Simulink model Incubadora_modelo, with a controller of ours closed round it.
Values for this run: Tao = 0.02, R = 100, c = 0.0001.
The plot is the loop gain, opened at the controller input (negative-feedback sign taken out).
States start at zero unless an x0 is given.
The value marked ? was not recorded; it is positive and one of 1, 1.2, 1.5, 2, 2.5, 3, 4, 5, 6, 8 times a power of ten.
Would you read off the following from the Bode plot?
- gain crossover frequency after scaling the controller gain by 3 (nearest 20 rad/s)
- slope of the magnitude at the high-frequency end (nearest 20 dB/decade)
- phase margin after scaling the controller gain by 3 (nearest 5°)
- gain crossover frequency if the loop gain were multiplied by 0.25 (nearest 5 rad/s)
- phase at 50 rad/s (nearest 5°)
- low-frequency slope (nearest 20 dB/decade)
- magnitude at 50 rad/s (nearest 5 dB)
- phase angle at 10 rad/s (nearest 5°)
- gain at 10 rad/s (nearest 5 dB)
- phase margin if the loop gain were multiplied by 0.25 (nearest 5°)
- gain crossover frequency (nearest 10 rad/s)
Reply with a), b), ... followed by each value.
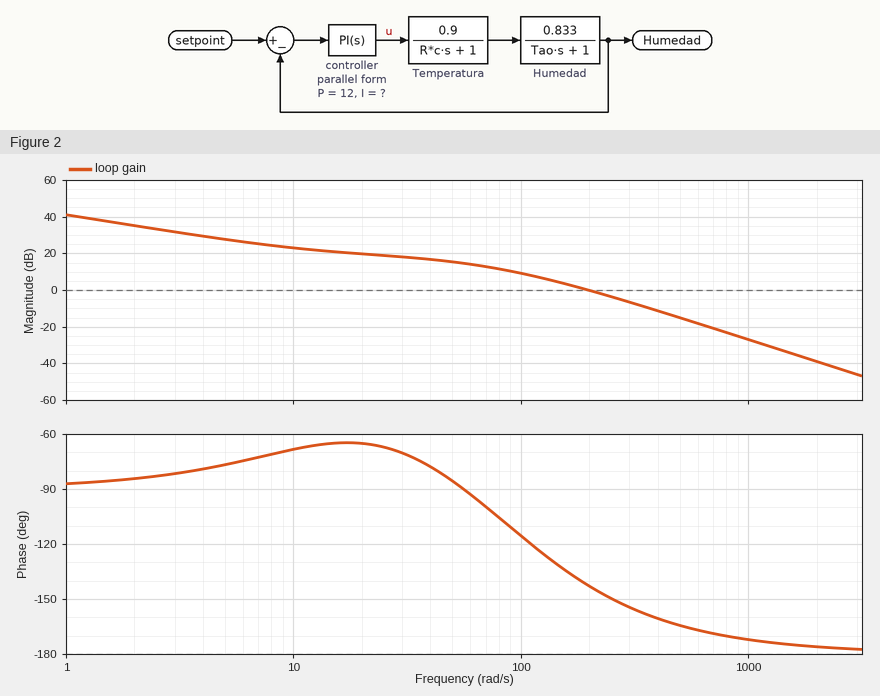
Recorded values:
a) 360 rad/s
b) -40 dB/decade
c) 20°
d) 75 rad/s
e) -85°
f) -20 dB/decade
g) 15 dB
h) -70°
i) 25 dB
j) 75°
k) 200 rad/s
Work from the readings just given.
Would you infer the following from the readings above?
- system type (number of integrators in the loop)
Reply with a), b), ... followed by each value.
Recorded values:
a) 1
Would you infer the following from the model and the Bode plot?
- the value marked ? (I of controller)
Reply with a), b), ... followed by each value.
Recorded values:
a) 150
